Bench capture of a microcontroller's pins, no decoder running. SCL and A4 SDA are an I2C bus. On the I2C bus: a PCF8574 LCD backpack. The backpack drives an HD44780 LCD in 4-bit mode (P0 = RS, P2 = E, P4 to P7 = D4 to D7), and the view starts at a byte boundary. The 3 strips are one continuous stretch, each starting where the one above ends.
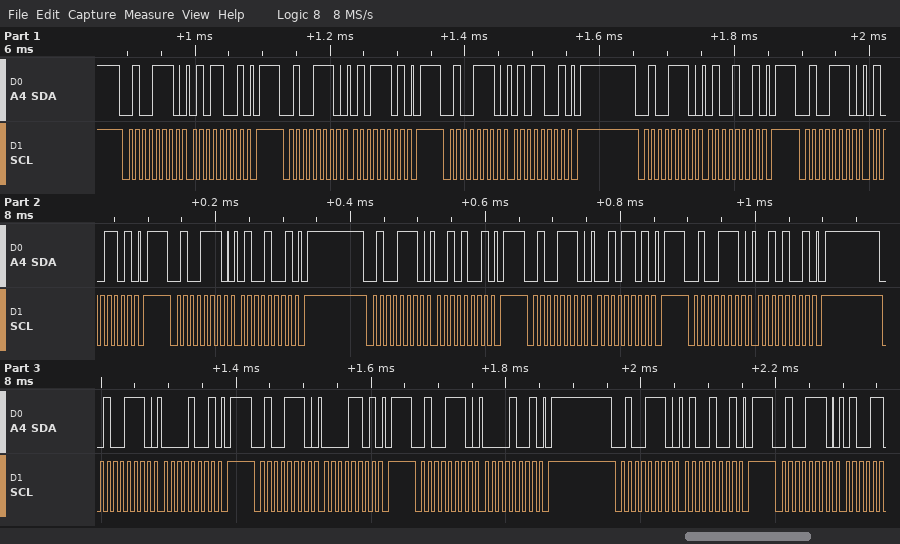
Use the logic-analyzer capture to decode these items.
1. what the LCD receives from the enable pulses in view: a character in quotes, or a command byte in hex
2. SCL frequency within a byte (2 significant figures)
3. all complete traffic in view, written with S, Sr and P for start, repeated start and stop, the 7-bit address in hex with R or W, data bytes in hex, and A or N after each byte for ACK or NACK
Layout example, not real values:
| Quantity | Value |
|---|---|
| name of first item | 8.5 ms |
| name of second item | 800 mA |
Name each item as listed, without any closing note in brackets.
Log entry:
| Quantity | Value |
|---|---|
| what the LCD receives from the enable pulses in view: a character in quotes, or a command byte in hex | 'T' ' ' |
| SCL frequency within a byte | 100 kHz |
| all complete traffic in view, written with S, Sr and P for start, repeated start and stop, the 7-bit address in hex with R or W, data bytes in hex, and A or N after each byte for ACK or NACK | S 27W A 59 A P S 27W A 5D A P S 27W A 59 A P S 27W A 49 A P S 27W A 4D A P S 27W A 49 A P S 27W A 29 A P S 27W A 2D A P S 27W A 29 A P S 27W A 09 A P S 27W A 0D A P S 27W A 09 A P S 27W A 49 A P S 27W A |
